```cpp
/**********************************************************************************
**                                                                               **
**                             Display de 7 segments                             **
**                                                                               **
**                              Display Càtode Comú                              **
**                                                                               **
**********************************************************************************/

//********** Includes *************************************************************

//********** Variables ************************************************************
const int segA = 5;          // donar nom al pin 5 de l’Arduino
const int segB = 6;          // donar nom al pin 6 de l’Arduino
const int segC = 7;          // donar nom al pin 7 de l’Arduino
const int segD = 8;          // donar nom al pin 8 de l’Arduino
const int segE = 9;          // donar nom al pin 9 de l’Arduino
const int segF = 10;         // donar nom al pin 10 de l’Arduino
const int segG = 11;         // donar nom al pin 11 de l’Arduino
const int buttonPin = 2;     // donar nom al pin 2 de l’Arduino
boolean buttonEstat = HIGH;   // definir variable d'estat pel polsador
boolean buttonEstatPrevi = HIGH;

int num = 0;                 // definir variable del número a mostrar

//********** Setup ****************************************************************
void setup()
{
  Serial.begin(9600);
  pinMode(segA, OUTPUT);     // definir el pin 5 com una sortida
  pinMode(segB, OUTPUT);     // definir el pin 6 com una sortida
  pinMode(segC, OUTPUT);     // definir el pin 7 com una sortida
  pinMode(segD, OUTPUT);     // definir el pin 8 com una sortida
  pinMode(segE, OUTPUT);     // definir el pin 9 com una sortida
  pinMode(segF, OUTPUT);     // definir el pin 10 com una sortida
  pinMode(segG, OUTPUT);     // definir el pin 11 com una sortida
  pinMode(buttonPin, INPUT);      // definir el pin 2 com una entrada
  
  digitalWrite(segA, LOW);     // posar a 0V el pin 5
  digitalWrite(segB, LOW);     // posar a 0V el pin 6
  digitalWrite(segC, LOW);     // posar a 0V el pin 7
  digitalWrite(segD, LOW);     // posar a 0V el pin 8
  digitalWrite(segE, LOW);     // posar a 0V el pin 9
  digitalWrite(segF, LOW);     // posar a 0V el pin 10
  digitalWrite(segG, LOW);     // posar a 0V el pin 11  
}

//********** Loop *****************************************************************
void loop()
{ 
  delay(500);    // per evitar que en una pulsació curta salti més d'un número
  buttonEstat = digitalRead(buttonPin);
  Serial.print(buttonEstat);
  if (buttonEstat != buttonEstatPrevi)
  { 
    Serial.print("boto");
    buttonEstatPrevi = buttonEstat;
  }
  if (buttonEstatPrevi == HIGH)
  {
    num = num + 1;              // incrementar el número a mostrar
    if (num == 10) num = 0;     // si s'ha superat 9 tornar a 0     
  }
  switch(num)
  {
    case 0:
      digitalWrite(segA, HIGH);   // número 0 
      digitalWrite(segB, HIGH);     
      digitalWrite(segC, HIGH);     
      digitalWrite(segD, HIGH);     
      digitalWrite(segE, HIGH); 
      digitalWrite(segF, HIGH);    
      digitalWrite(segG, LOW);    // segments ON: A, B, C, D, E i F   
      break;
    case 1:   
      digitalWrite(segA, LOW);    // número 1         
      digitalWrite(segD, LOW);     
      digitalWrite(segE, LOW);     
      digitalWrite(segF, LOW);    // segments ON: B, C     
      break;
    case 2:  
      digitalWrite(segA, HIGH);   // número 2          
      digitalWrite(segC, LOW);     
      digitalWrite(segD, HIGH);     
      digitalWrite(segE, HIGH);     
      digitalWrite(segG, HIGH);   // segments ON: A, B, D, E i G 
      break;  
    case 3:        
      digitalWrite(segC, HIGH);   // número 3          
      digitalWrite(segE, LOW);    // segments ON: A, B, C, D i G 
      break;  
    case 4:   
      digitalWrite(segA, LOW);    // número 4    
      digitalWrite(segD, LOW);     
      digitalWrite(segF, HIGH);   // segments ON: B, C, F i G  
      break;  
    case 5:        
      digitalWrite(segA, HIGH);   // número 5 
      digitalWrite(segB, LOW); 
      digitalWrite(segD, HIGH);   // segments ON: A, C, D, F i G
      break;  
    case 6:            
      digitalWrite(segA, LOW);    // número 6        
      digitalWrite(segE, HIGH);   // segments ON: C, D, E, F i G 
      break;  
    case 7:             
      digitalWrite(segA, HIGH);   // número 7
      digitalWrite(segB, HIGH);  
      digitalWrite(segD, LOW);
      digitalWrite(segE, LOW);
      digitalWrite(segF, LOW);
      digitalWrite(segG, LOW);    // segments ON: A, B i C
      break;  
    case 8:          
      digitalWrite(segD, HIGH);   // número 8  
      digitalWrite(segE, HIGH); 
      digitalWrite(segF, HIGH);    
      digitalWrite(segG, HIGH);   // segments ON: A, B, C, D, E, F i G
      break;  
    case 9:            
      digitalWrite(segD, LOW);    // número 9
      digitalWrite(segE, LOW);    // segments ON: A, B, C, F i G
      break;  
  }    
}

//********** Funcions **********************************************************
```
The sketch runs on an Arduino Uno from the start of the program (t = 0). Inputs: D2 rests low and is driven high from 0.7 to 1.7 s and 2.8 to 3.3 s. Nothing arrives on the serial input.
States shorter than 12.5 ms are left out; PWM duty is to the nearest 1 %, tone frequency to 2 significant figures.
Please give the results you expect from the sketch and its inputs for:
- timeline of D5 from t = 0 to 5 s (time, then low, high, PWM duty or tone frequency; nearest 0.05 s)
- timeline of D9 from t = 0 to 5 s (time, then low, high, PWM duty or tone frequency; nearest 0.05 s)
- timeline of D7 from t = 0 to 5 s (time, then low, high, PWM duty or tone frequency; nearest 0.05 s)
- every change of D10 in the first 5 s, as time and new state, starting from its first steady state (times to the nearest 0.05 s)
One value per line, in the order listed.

0 s low; 0.5 s high; 1 s low; 1.5 s high
0 s low; 0.5 s high; 1 s low; 1.5 s high; 3 s low
0 s low; 0.5 s high; 1.5 s low; 3 s high
0 s low; 0.5 s high; 1 s low
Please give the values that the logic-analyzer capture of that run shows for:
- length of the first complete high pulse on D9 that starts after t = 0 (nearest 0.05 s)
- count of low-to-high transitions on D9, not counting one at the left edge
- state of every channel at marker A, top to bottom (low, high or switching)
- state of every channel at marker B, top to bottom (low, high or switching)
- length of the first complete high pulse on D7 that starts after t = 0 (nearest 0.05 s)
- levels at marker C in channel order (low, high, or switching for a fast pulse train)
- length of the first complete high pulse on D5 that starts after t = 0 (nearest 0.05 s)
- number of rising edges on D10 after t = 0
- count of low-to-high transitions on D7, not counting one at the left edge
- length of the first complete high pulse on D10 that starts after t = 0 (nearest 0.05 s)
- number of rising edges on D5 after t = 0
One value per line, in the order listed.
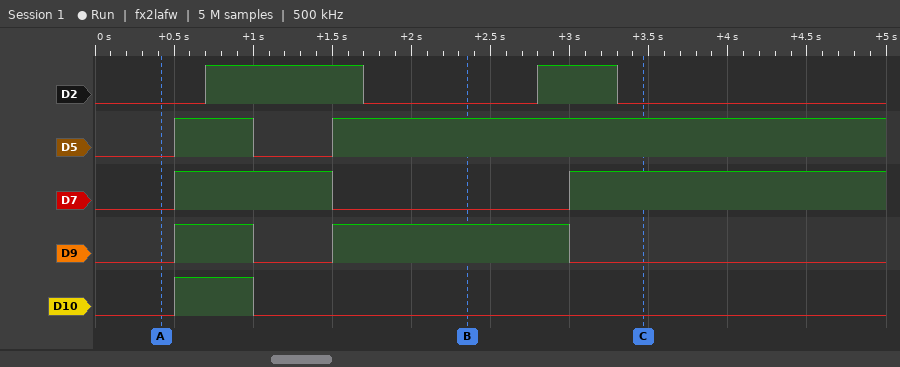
0.50 s
2
D2 low, D5 low, D7 low, D9 low, D10 low
D2 low, D5 high, D7 low, D9 high, D10 low
1.00 s
D2 low, D5 high, D7 high, D9 low, D10 low
0.50 s
1
2
0.50 s
2
